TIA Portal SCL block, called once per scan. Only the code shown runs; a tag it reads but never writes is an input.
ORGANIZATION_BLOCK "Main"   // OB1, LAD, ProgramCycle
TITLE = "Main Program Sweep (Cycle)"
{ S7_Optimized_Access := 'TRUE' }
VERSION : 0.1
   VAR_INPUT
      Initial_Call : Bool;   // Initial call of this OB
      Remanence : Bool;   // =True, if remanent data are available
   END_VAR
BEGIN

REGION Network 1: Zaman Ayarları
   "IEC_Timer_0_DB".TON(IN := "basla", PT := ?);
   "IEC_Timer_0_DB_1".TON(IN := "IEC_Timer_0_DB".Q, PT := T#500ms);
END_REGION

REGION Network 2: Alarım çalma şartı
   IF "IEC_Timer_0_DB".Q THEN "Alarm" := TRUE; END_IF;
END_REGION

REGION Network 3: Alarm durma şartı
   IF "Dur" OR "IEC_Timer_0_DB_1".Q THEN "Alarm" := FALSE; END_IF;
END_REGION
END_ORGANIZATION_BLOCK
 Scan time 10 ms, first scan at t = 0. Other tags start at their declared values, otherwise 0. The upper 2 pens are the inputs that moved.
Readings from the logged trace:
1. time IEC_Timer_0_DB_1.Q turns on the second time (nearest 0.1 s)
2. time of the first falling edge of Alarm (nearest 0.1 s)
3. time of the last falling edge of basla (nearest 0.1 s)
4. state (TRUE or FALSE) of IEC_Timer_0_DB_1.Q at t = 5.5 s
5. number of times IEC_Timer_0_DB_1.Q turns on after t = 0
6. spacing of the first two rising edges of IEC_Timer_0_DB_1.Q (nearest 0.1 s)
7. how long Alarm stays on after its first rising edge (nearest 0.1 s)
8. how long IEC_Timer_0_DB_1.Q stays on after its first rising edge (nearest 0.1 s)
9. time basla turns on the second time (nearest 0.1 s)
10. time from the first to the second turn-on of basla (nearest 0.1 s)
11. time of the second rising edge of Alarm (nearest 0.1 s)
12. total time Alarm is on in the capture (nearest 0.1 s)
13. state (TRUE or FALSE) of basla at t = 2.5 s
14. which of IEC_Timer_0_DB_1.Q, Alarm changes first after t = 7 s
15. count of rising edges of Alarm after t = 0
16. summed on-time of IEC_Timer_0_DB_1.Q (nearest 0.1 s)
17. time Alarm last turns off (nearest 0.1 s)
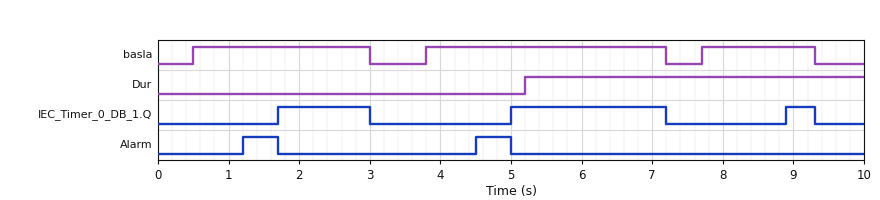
5.0 s
1.7 s
9.3 s
TRUE
3
3.3 s
0.5 s
1.3 s
3.8 s
3.3 s
4.5 s
1.0 s
TRUE
IEC_Timer_0_DB_1.Q
2
3.9 s
5.0 s
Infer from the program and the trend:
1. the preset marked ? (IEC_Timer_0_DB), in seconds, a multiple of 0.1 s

0.7 s
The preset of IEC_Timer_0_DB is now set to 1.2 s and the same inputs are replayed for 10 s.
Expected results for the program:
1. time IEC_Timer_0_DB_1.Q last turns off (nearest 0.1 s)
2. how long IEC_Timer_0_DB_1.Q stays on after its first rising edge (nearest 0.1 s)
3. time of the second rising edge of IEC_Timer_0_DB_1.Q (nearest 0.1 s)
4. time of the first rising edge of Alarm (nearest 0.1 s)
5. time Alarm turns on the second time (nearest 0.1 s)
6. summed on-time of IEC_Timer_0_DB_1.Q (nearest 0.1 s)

7.2 s
0.8 s
5.5 s
1.7 s
5.0 s
2.5 s
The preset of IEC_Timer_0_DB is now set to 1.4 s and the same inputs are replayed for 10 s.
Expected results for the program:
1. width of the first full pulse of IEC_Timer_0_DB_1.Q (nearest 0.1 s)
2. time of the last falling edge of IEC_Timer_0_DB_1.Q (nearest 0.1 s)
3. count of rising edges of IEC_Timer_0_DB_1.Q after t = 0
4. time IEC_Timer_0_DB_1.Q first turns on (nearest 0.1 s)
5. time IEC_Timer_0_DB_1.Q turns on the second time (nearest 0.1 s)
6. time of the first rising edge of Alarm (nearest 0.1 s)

0.6 s
7.2 s
2
2.4 s
5.7 s
1.9 s
